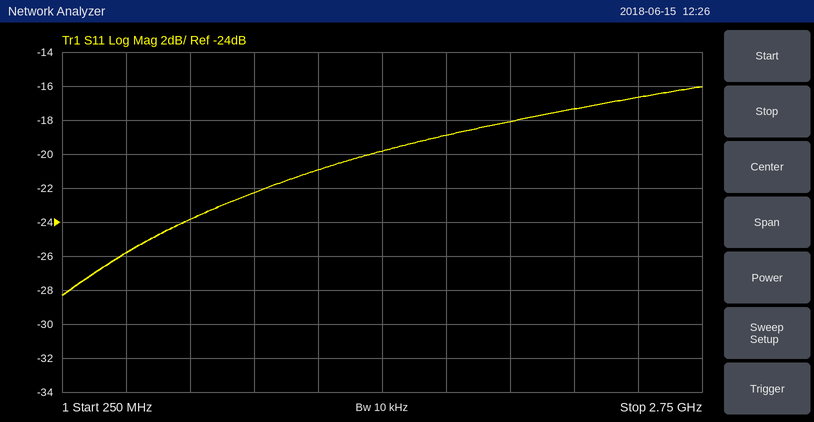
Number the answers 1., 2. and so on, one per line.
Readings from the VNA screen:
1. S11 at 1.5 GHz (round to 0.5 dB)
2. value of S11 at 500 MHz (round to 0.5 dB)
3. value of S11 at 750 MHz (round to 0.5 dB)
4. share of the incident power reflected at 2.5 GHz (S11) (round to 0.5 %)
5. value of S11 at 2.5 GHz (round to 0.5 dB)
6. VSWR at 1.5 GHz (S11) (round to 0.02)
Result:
1. -20.0 dB
2. -26.0 dB
3. -24.0 dB
4. 2.0 %
5. -16.5 dB
6. 1.22
